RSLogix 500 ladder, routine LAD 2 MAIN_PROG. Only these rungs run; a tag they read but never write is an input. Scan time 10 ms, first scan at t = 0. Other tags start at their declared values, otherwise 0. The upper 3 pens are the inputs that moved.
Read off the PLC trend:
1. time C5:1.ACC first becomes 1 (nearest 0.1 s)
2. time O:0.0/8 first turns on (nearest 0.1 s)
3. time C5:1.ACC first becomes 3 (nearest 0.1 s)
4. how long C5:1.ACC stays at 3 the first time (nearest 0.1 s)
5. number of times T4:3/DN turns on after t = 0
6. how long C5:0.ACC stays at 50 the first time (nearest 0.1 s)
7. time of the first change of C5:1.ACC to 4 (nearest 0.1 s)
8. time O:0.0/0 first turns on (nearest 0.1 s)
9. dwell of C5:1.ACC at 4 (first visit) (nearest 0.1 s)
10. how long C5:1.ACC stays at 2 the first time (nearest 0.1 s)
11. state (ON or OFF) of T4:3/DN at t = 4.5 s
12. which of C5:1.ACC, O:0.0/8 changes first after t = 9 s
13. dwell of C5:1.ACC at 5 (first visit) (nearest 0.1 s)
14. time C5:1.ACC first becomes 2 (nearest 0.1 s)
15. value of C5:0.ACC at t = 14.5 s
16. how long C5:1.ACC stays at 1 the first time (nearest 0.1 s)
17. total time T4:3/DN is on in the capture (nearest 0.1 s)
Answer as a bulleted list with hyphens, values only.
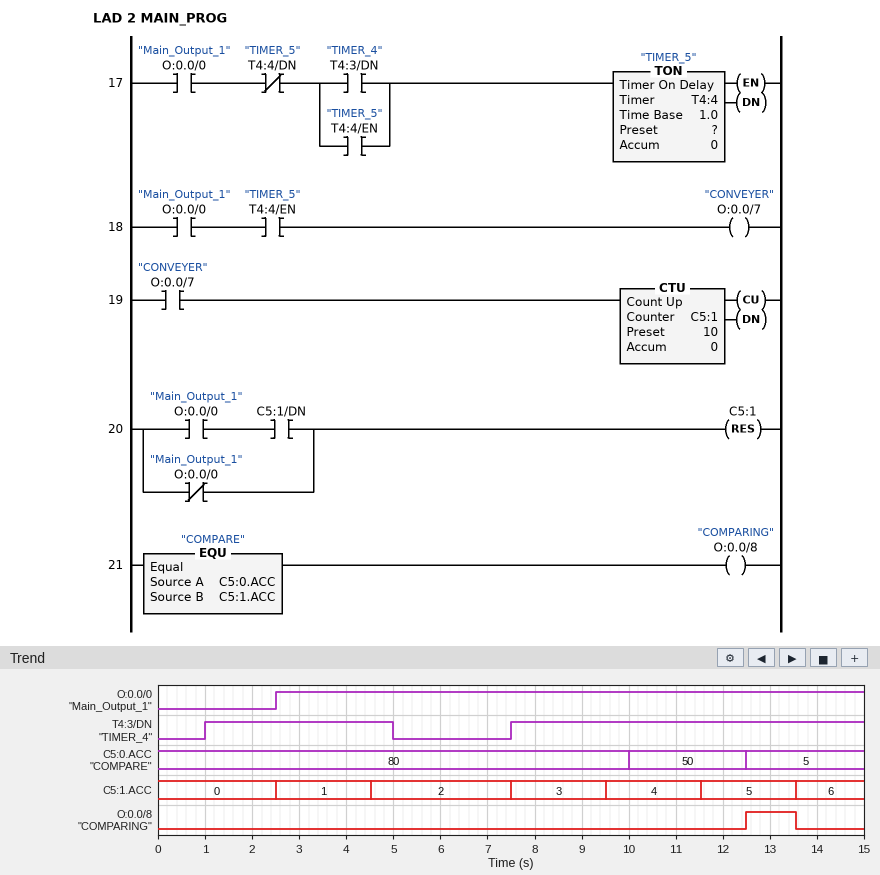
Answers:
- 2.5 s
- 12.5 s
- 7.5 s
- 2.0 s
- 2
- 2.5 s
- 9.5 s
- 2.5 s
- 2.0 s
- 3.0 s
- ON
- C5:1.ACC
- 2.0 s
- 4.5 s
- 5
- 2.0 s
- 11.5 s
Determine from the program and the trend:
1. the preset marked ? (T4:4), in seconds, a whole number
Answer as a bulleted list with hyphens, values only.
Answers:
- 2 s
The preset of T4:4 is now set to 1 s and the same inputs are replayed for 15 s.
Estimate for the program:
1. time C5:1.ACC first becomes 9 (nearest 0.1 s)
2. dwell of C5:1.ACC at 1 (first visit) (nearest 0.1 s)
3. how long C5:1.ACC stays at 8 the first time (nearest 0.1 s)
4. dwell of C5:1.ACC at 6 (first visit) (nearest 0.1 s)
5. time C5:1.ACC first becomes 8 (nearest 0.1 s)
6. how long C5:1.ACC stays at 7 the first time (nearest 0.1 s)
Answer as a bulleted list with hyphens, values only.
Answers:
- 12.6 s
- 1.0 s
- 1.0 s
- 1.0 s
- 11.6 s
- 1.0 s
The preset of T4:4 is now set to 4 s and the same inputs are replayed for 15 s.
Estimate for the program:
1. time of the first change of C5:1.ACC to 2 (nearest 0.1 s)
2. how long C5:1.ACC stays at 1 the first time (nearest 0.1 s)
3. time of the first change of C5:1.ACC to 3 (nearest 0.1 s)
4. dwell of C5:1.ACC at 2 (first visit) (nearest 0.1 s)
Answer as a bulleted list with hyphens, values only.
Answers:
- 7.5 s
- 5.0 s
- 11.5 s
- 4.0 s
